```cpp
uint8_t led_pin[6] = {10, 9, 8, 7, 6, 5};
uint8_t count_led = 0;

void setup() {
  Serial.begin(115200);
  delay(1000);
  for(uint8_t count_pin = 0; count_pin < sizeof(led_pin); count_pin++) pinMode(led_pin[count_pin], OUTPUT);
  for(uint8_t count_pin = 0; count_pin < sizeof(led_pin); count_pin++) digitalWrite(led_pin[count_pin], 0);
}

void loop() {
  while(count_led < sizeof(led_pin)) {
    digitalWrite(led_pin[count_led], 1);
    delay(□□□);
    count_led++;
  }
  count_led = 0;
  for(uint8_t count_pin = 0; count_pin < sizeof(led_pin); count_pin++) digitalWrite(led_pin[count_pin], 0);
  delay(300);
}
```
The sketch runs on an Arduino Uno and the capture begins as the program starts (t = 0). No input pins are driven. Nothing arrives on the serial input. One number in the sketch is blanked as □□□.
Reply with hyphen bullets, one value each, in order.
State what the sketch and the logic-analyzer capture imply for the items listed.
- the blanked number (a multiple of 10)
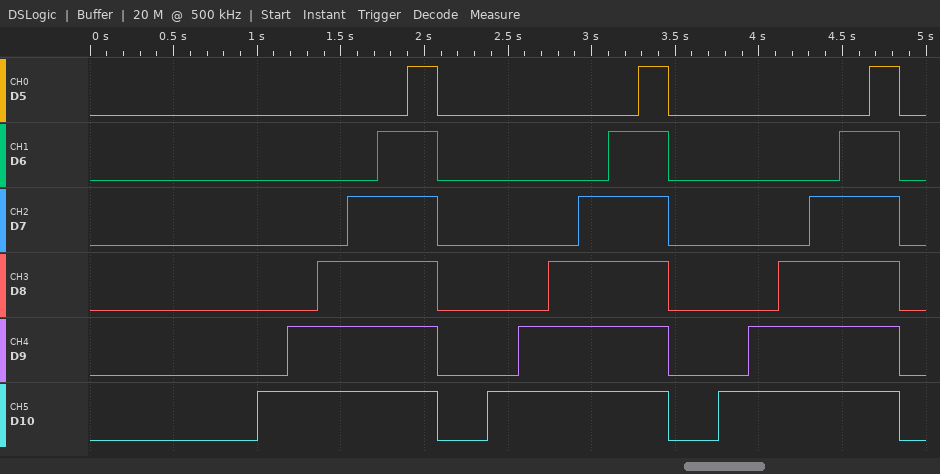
- 180
